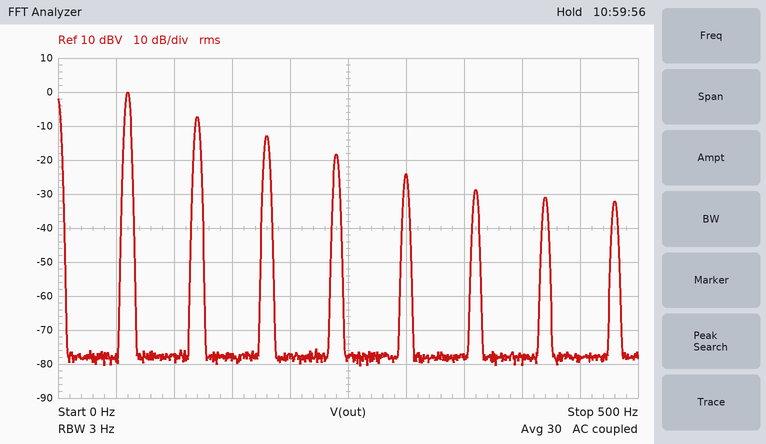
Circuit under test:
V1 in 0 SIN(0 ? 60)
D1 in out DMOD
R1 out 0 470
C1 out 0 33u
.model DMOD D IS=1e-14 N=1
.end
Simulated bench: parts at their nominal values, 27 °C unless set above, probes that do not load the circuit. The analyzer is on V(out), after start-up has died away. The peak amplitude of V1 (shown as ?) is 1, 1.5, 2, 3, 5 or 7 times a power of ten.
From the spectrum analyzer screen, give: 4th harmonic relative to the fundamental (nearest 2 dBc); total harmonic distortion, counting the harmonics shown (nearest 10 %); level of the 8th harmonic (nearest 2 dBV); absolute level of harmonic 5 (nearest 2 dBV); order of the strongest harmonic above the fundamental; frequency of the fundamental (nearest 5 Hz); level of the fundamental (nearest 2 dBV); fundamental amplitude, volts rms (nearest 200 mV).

-18 dBc
50 %
-32 dBV
-24 dBV
2
60 Hz
0 dBV
1.0 V
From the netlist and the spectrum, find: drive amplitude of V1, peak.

7 V
